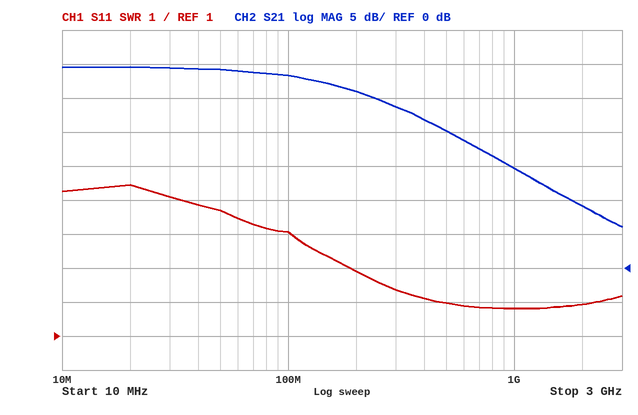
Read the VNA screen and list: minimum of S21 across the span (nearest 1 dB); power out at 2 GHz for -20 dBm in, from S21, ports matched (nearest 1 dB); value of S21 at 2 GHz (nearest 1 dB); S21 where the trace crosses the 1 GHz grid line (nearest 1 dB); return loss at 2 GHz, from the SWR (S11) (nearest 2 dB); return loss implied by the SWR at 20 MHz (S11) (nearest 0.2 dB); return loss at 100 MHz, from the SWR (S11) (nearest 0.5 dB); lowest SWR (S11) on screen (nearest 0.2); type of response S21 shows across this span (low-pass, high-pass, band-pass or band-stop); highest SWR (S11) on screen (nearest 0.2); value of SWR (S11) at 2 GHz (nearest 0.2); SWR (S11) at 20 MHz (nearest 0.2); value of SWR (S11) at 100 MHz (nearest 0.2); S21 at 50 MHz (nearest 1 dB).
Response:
6 dB
-11 dBm
9 dB
15 dB
10 dB
3.2 dB
4.5 dB
1.8
low-pass
5.4
2.0
5.4
4.0
29 dB
